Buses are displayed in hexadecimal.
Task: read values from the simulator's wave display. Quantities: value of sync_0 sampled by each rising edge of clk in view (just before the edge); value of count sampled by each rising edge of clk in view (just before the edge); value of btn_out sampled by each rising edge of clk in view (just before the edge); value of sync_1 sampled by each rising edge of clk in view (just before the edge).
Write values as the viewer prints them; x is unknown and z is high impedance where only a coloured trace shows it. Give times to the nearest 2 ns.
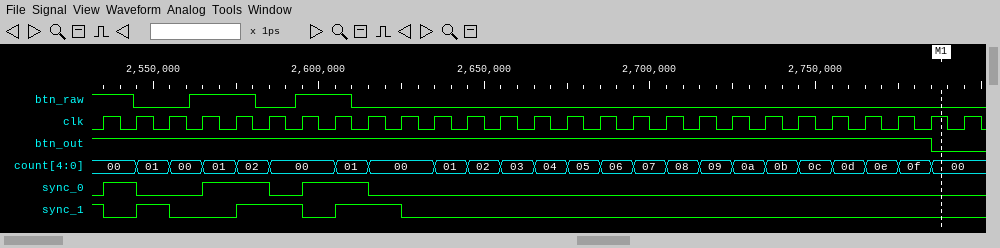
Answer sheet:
0 1 0 0 1 1 0 1 1 0 0 0 0 0 0 0 0 0 0 0 0 0 0 0 0 0 0
00, 00, 01, 00, 01, 02, 00, 00, 01, 00, 00, 01, 02, 03, 04, 05, 06, 07, 08, 09, 0a, 0b, 0c, 0d, 0e, 0f, 00
1 1 1 1 1 1 1 1 1 1 1 1 1 1 1 1 1 1 1 1 1 1 1 1 1 1 0
1 0 1 0 0 1 1 0 1 1 0 0 0 0 0 0 0 0 0 0 0 0 0 0 0 0 0
